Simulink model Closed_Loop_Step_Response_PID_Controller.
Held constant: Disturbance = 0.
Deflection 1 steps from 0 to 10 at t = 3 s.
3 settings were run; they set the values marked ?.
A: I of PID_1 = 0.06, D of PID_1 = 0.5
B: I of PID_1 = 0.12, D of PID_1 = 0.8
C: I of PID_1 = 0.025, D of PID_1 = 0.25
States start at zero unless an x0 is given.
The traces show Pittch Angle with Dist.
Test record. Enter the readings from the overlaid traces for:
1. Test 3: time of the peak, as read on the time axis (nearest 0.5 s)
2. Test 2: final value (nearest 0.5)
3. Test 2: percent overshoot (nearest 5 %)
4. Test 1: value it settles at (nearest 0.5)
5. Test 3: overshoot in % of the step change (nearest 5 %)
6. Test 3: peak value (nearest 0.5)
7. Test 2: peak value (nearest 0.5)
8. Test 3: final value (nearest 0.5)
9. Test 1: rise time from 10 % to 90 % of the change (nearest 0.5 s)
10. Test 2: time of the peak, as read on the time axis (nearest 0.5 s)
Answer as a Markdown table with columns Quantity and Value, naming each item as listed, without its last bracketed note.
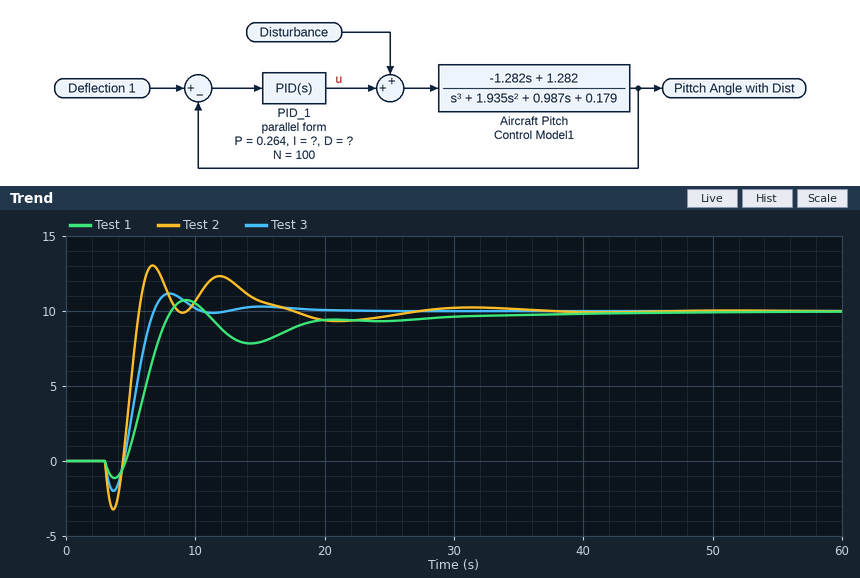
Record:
| Quantity | Value |
|---|---|
| Test 3: time of the peak, as read on the time axis | 8.0 s |
| Test 2: final value | 10.0 |
| Test 2: percent overshoot | 30 % |
| Test 1: value it settles at | 10.0 |
| Test 3: overshoot in % of the step change | 10 % |
| Test 3: peak value | 11.0 |
| Test 2: peak value | 13.0 |
| Test 3: final value | 10.0 |
| Test 1: rise time from 10 % to 90 % of the change | 2.5 s |
| Test 2: time of the peak, as read on the time axis | 6.5 s |
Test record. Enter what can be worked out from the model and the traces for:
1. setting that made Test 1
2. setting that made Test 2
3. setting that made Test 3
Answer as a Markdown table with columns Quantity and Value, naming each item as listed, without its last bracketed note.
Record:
| Quantity | Value |
|---|---|
| setting that made Test 1 | C |
| setting that made Test 2 | B |
| setting that made Test 3 | A |
